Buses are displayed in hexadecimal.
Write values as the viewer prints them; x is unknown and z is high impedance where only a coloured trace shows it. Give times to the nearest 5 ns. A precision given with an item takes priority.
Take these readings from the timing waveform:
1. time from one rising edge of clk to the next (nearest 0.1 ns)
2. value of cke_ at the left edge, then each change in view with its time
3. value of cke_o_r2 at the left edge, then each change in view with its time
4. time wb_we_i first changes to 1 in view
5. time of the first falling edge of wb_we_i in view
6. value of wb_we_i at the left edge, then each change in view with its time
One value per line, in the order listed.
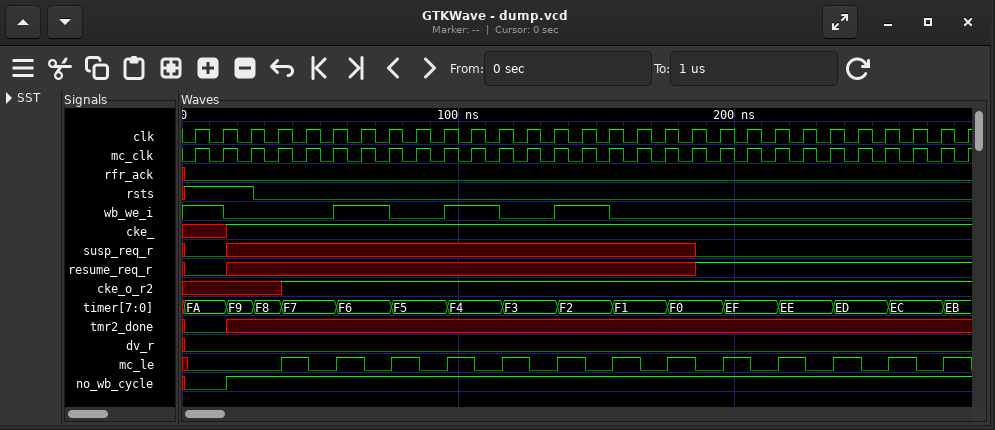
10 ns
x, 1 at 15 ns
x, 1 at 35 ns
55 ns
15 ns
1, 0 at 15 ns, 1 at 55 ns, 0 at 75 ns, 1 at 95 ns, 0 at 115 ns, 1 at 135 ns, 0 at 155 ns
